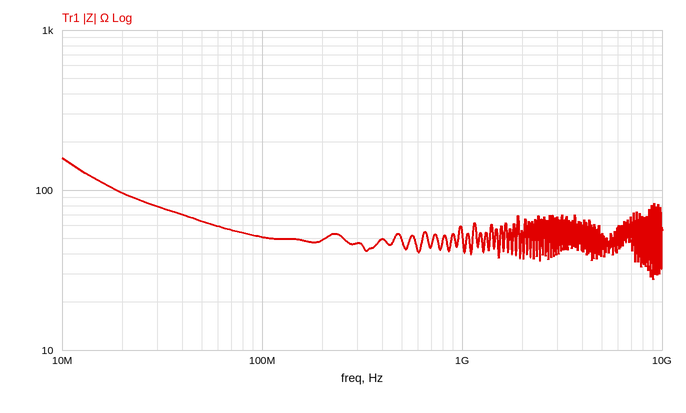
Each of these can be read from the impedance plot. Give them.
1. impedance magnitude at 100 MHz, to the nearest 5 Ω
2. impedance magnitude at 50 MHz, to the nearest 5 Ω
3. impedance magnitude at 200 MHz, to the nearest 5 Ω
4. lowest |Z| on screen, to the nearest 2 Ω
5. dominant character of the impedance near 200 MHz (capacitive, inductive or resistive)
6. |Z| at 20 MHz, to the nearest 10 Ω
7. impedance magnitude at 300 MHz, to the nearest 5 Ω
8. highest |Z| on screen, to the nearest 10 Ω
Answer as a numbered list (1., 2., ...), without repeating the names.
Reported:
1. 50 Ω
2. 65 Ω
3. 50 Ω
4. 28 Ω
5. resistive
6. 100 Ω
7. 45 Ω
8. 160 Ω
